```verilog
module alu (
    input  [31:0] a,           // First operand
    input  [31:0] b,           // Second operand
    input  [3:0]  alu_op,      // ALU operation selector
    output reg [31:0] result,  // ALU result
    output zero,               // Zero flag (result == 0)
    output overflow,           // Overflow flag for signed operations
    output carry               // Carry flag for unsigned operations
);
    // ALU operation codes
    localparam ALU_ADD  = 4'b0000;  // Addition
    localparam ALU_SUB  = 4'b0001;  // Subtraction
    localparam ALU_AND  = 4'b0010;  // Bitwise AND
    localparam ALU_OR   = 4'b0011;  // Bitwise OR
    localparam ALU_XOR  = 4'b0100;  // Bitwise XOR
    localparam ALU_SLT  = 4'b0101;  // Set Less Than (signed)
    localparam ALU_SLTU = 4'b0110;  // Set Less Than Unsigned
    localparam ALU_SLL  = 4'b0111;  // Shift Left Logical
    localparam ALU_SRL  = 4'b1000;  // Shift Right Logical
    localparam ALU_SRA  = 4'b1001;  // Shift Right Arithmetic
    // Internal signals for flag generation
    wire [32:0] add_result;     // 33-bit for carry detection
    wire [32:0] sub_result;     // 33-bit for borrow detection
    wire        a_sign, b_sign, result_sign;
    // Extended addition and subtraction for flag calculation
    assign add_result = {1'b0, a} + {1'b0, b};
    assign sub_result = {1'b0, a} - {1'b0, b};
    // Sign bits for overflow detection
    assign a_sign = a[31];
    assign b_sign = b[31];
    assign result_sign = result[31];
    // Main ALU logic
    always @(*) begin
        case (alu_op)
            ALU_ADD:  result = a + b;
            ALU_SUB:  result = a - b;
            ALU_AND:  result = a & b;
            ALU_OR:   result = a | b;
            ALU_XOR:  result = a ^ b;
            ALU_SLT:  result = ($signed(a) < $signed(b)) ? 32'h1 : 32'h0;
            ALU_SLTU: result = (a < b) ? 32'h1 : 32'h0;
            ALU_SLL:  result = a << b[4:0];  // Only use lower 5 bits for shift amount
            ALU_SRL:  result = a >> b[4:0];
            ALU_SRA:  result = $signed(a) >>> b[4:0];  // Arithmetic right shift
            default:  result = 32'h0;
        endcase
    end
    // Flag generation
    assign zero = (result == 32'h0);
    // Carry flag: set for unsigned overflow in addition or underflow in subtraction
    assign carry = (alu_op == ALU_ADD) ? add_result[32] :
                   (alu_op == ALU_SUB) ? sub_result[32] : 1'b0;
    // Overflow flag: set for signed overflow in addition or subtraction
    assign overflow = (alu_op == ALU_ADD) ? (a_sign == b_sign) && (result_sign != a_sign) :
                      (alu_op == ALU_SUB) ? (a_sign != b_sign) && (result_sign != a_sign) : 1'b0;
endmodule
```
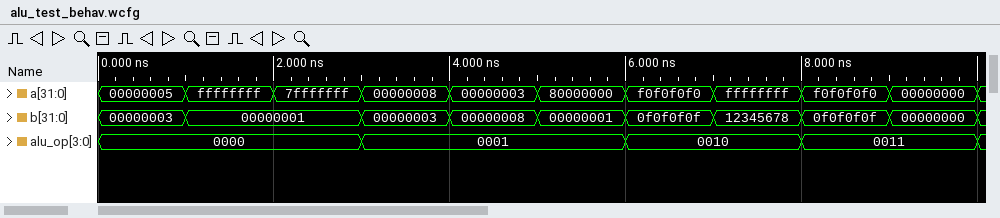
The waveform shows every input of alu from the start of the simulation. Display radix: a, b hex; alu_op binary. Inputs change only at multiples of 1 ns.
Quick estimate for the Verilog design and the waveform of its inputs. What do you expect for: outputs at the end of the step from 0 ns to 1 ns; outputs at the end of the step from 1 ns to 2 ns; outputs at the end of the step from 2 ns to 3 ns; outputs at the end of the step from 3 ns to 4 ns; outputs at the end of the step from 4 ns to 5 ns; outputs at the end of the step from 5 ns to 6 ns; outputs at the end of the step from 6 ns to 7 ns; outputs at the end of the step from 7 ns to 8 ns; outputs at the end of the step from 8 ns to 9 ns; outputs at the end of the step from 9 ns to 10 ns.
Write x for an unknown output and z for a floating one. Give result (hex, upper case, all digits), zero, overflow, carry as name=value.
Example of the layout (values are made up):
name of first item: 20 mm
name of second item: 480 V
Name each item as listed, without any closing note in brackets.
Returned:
outputs at the end of the step from 0 ns to 1 ns: result=00000008, zero=0, overflow=0, carry=0
outputs at the end of the step from 1 ns to 2 ns: result=00000000, zero=1, overflow=0, carry=1
outputs at the end of the step from 2 ns to 3 ns: result=80000000, zero=0, overflow=1, carry=0
outputs at the end of the step from 3 ns to 4 ns: result=00000005, zero=0, overflow=0, carry=0
outputs at the end of the step from 4 ns to 5 ns: result=FFFFFFFB, zero=0, overflow=0, carry=1
outputs at the end of the step from 5 ns to 6 ns: result=7FFFFFFF, zero=0, overflow=1, carry=0
outputs at the end of the step from 6 ns to 7 ns: result=00000000, zero=1, overflow=0, carry=0
outputs at the end of the step from 7 ns to 8 ns: result=12345678, zero=0, overflow=0, carry=0
outputs at the end of the step from 8 ns to 9 ns: result=FFFFFFFF, zero=0, overflow=0, carry=0
outputs at the end of the step from 9 ns to 10 ns: result=00000000, zero=1, overflow=0, carry=0
